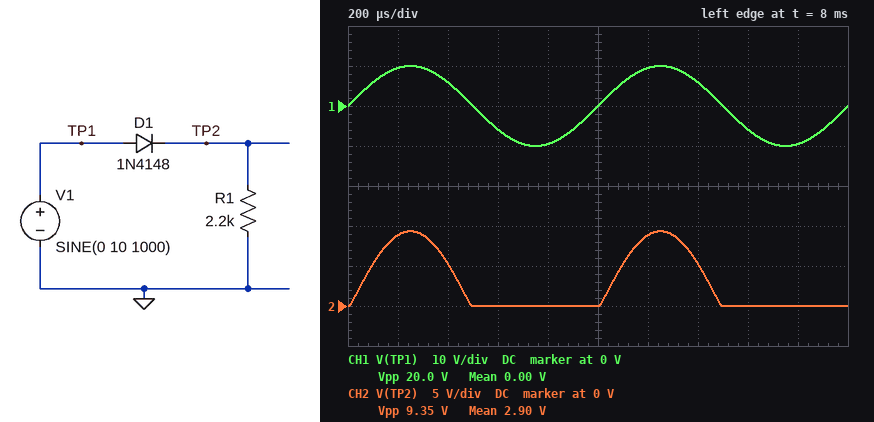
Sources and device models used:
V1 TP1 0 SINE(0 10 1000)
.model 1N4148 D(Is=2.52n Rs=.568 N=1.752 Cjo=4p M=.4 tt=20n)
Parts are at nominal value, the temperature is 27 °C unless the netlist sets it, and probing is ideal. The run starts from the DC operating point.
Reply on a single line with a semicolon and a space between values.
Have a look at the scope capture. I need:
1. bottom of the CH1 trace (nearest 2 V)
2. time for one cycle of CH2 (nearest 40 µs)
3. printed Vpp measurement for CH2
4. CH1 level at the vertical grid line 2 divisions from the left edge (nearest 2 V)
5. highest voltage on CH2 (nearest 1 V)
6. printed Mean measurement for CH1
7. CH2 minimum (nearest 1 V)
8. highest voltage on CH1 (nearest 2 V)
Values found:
-10 V; 1.00 ms; 9.35 V; 6 V; 9 V; 0.00 V; 0 V; 10 V
